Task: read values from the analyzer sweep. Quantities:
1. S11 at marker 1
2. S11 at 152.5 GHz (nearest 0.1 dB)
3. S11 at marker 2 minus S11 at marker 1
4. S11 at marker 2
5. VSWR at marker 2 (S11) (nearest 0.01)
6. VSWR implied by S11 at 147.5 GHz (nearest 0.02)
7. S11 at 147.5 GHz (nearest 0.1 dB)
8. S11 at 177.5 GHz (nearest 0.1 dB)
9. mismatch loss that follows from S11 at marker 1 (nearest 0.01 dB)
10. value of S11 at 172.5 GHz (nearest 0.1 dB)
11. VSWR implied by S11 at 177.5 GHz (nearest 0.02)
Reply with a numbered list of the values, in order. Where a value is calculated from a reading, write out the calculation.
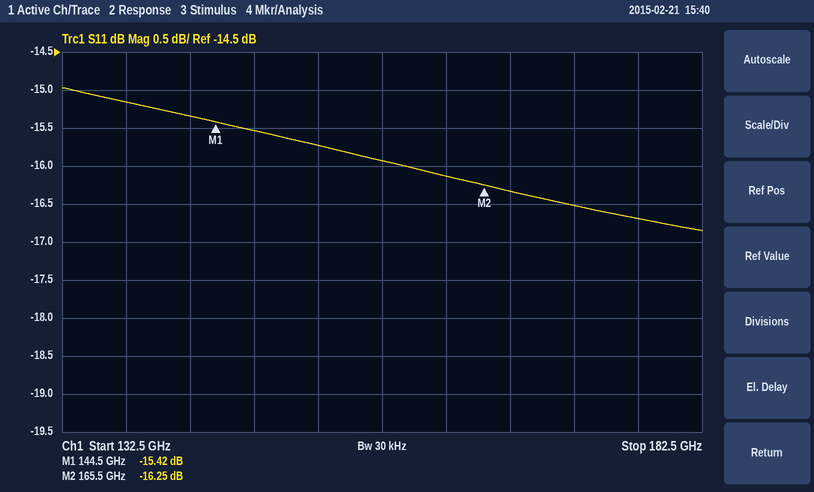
1. -15.42 dB
2. -15.7 dB
3. -16.25 − (-15.42) = -0.83 dB
4. -16.25 dB
5. (1 + 0.1540)/(1 − 0.1540) ≈ 1.36
6. |Γ| = 10^(-15.5/20) = 0.1679; VSWR = (1 + 0.1679)/(1 − 0.1679) ≈ 1.40
7. -15.5 dB
8. -16.7 dB
9. −10 log10(1 − 10^(-15.42/10)) ≈ 0.13 dB
10. -16.5 dB
11. |Γ| = 10^(-16.7/20) = 0.1462; VSWR = (1 + 0.1462)/(1 − 0.1462) ≈ 1.34
